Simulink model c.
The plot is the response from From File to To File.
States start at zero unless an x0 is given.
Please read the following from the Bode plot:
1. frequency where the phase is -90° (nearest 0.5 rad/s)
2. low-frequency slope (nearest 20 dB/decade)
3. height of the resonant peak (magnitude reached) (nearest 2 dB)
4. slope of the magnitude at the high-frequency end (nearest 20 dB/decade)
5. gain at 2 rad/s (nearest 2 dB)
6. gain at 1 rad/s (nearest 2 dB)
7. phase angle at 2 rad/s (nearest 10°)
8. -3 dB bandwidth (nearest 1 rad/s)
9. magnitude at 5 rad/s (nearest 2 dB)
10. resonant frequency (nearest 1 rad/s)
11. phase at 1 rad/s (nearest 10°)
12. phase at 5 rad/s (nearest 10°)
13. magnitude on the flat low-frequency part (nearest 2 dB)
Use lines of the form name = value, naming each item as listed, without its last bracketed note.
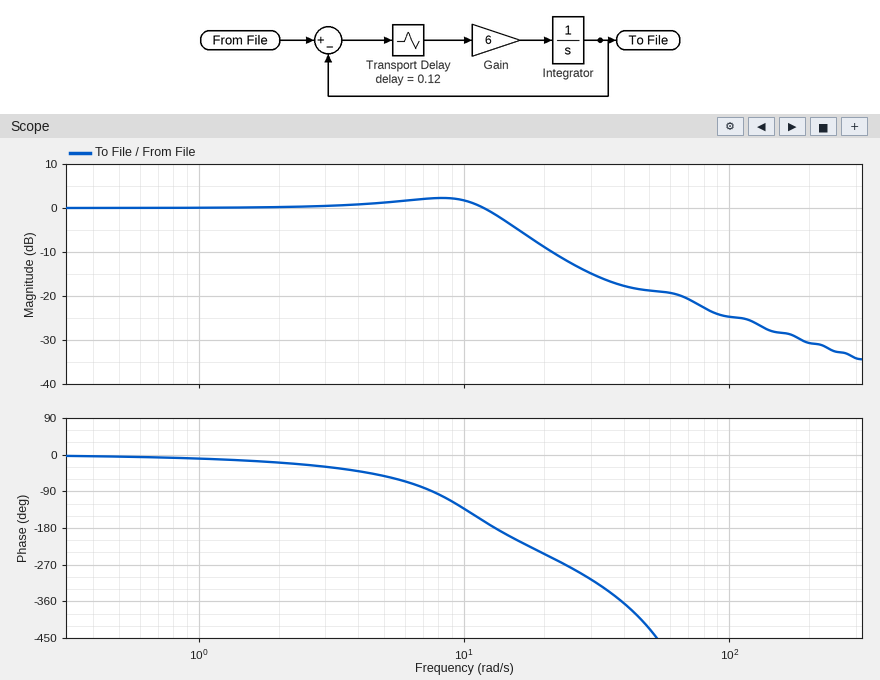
frequency where the phase is -90° = 7.5 rad/s
low-frequency slope = 0 dB/decade
height of the resonant peak (magnitude reached) = 2 dB
slope of the magnitude at the high-frequency end = -20 dB/decade
gain at 2 rad/s = 0 dB
gain at 1 rad/s = 0 dB
phase angle at 2 rad/s = -20°
-3 dB bandwidth = 14 rad/s
magnitude at 5 rad/s = 2 dB
resonant frequency = 8 rad/s
phase at 1 rad/s = -10°
phase at 5 rad/s = -50°
magnitude on the flat low-frequency part = 0 dB
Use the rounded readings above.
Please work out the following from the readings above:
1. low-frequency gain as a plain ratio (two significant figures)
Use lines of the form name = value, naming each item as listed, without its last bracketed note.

low-frequency gain as a plain ratio = 1.0
